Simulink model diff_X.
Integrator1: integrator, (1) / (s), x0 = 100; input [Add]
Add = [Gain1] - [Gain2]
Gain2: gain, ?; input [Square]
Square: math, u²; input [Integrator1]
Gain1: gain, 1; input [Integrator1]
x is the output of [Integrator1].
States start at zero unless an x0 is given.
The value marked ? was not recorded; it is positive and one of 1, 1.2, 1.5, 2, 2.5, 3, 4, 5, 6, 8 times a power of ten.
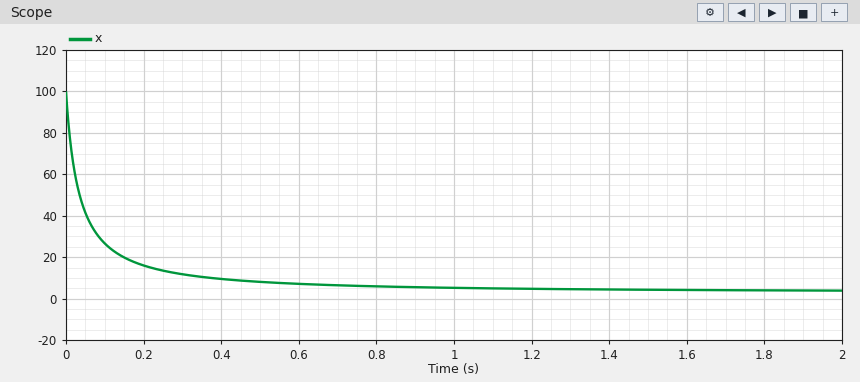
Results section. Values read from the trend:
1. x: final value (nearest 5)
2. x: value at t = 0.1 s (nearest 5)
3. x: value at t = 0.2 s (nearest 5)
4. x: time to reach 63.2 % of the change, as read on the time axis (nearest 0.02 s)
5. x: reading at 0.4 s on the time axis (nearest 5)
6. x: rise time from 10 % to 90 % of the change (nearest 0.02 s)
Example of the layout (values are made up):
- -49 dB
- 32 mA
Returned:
- 5
- 25
- 15
- 0.06 s
- 10
- 0.26 s
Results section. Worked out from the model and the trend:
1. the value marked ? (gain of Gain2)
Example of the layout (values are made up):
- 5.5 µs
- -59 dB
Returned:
- 0.3
